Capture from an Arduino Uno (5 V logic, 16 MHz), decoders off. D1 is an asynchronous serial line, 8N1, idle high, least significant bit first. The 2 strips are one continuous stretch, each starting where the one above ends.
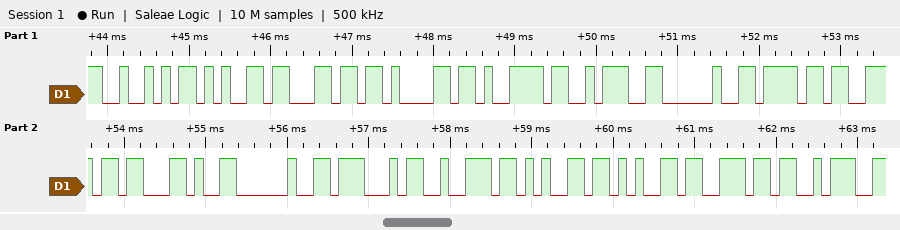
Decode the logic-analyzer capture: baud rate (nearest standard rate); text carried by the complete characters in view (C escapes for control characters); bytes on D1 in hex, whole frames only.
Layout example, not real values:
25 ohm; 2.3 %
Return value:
9600 baud; "Relay: on, Green:"; 52 65 6C 61 79 3A 20 6F 6E 2C 20 47 72 65 65 6E 3A
